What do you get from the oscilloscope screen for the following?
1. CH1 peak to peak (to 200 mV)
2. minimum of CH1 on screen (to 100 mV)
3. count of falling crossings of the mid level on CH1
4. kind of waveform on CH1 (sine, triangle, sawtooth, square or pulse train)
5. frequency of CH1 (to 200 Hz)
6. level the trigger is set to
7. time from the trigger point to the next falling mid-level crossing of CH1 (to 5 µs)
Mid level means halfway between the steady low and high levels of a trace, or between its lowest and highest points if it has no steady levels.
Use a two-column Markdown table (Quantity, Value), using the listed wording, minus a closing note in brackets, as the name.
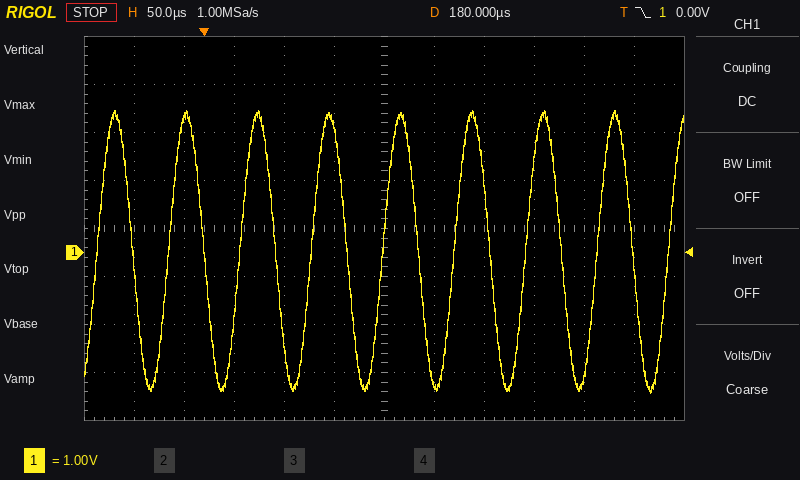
| Quantity | Value |
|---|---|
| CH1 peak to peak | 5.8 V |
| minimum of CH1 on screen | -2.9 V |
| count of falling crossings of the mid level on CH1 | 8 |
| kind of waveform on CH1 | sine |
| frequency of CH1 | 14.0 kHz |
| level the trigger is set to | 0.00 V |
| time from the trigger point to the next falling mid-level crossing of CH1 | 70 µs |
